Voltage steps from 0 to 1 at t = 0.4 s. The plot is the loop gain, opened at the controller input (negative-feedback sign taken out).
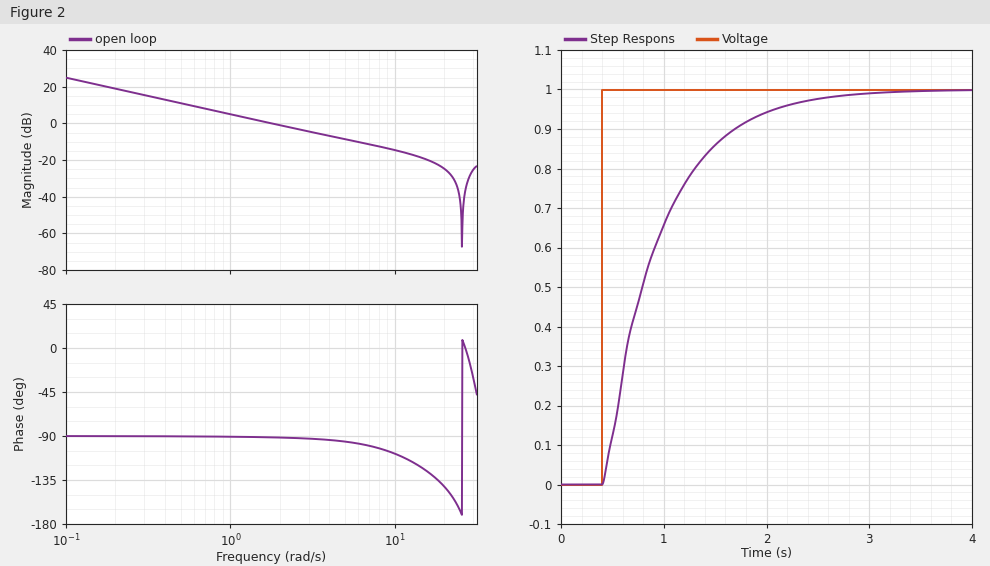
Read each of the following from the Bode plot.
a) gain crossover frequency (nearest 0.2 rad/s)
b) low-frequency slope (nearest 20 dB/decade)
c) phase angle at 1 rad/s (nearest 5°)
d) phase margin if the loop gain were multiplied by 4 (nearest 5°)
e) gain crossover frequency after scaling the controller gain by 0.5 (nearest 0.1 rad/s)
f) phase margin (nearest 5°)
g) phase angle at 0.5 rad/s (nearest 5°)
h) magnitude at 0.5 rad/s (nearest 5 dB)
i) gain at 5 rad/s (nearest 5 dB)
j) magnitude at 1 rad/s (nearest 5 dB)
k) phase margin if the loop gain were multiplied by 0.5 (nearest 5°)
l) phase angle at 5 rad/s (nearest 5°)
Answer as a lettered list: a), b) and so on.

a) 1.8 rad/s
b) -20 dB/decade
c) -90°
d) 80°
e) 0.9 rad/s
f) 90°
g) -90°
h) 10 dB
i) -10 dB
j) 5 dB
k) 90°
l) -95°
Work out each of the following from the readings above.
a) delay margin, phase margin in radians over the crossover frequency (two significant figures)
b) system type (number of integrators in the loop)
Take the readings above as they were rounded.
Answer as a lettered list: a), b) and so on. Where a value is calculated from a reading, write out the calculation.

a) 90 × π / 180 / 1.8 = 0.87 s
b) 1
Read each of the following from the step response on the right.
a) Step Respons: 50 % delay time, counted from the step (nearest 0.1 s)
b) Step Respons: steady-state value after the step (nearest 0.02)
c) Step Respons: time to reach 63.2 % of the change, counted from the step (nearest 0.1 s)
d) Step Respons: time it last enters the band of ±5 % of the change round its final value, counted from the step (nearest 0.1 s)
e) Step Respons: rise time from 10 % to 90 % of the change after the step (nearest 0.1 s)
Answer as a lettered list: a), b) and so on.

a) 0.4 s
b) 1.00
c) 0.6 s
d) 1.7 s
e) 1.2 s
